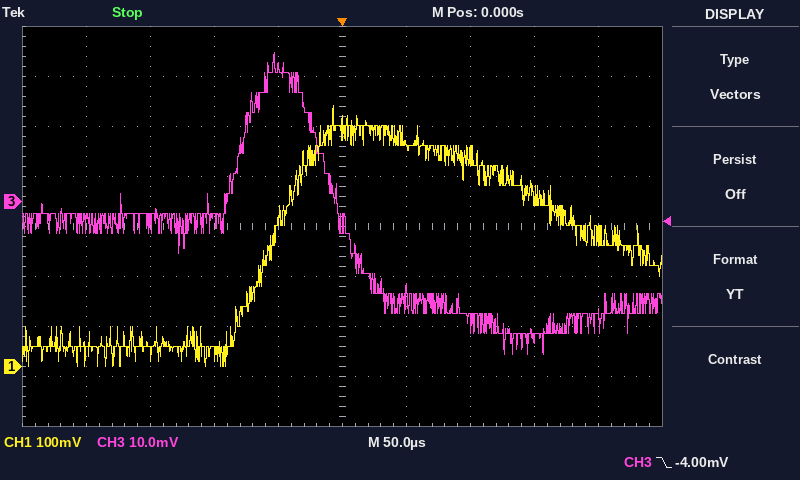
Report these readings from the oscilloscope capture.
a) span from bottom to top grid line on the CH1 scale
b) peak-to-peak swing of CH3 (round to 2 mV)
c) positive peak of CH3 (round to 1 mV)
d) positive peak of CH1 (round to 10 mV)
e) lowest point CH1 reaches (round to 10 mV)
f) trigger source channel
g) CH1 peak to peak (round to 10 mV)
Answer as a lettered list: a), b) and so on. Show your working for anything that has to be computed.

a) 800 mV
b) 60 mV
c) 30 mV
d) 520 mV
e) 0 mV
f) CH3
g) 520 mV − (0 mV) = 520 mV
